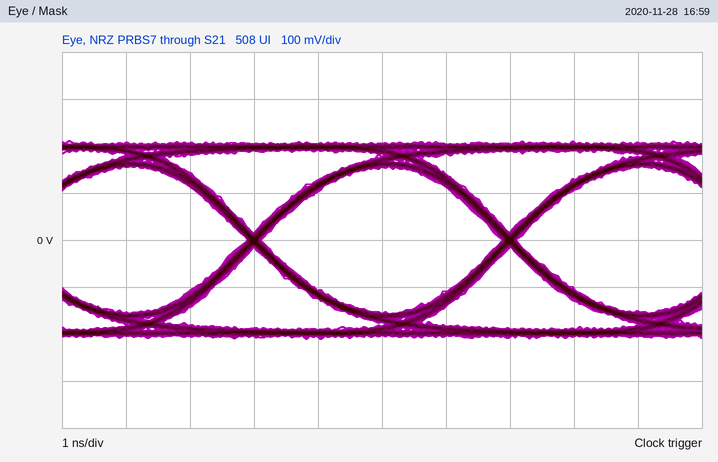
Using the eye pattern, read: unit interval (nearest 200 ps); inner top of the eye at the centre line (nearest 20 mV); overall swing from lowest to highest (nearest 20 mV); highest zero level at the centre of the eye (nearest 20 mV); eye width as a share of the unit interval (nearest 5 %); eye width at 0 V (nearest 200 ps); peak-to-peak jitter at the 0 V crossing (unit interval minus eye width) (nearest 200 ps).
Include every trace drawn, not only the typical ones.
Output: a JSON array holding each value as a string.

["4.0 ns", "160 mV", "420 mV", "-160 mV", "95 %", "3.8 ns", "200 ps"]
